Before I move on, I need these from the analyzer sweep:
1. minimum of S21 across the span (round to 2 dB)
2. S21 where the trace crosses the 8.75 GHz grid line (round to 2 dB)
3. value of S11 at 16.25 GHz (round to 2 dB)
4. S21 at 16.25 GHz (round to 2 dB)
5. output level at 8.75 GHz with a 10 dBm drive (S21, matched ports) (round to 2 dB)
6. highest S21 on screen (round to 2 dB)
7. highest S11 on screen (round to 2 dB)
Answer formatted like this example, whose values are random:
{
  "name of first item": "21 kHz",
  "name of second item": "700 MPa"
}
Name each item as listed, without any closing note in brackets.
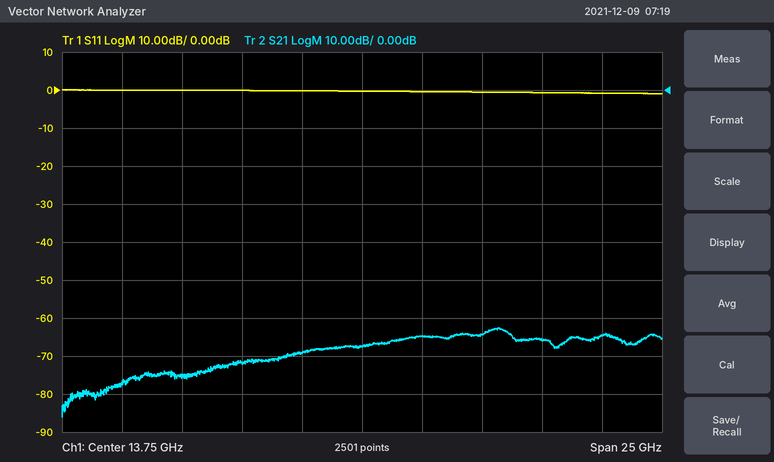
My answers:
{
  "minimum of S21 across the span": "-86 dB",
  "S21 where the trace crosses the 8.75 GHz grid line": "-72 dB",
  "value of S11 at 16.25 GHz": "0 dB",
  "S21 at 16.25 GHz": "-64 dB",
  "output level at 8.75 GHz with a 10 dBm drive (S21, matched ports)": "-62 dBm",
  "highest S21 on screen": "-62 dB",
  "highest S11 on screen": "0 dB"
}
